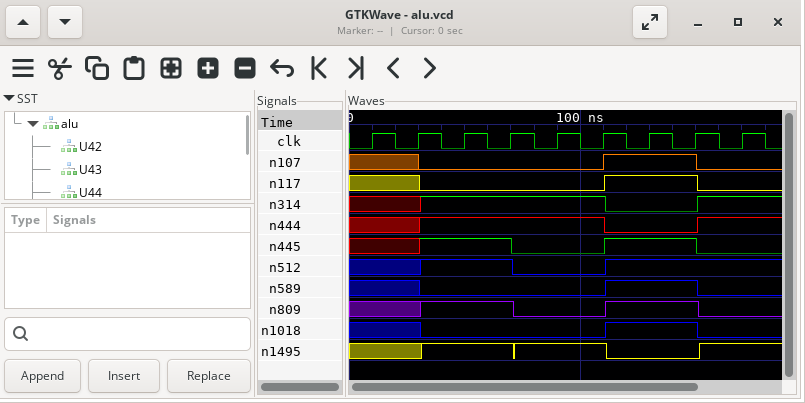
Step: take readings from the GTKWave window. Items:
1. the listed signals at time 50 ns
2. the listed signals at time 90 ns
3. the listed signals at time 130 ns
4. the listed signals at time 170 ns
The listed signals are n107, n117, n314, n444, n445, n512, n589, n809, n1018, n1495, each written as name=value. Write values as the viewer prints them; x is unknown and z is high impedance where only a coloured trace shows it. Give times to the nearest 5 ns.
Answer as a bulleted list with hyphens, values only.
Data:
- n107=0, n117=0, n314=1, n444=1, n445=1, n512=1, n589=0, n809=1, n1018=0, n1495=1
- n107=0, n117=0, n314=1, n444=1, n445=0, n512=0, n589=0, n809=0, n1018=0, n1495=1
- n107=1, n117=1, n314=0, n444=0, n445=1, n512=1, n589=1, n809=1, n1018=1, n1495=0
- n107=0, n117=0, n314=1, n444=1, n445=0, n512=1, n589=0, n809=0, n1018=0, n1495=1
